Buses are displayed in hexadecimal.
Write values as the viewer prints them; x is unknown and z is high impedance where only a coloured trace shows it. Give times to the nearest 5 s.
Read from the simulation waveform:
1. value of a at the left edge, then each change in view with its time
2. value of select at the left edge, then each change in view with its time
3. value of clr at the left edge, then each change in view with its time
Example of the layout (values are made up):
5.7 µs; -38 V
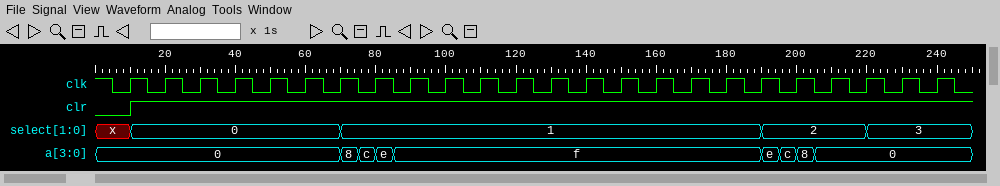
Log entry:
0, 8 at 70 s, c at 75 s, e at 80 s, f at 85 s, e at 190 s, c at 195 s, 8 at 200 s, 0 at 205 s; x, 0 at 10 s, 1 at 70 s, 2 at 190 s, 3 at 220 s; 0, 1 at 10 s
